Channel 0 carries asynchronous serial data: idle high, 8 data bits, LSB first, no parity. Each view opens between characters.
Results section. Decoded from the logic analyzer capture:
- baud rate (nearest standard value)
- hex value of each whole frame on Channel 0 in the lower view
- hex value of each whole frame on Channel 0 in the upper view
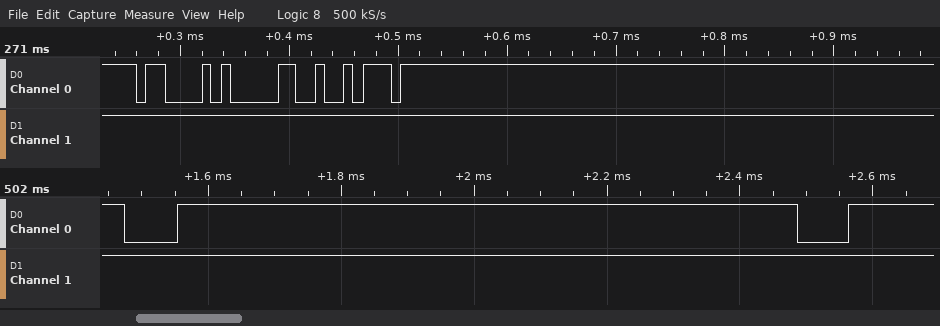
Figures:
115200 baud
00, 00
43, 30, BA
